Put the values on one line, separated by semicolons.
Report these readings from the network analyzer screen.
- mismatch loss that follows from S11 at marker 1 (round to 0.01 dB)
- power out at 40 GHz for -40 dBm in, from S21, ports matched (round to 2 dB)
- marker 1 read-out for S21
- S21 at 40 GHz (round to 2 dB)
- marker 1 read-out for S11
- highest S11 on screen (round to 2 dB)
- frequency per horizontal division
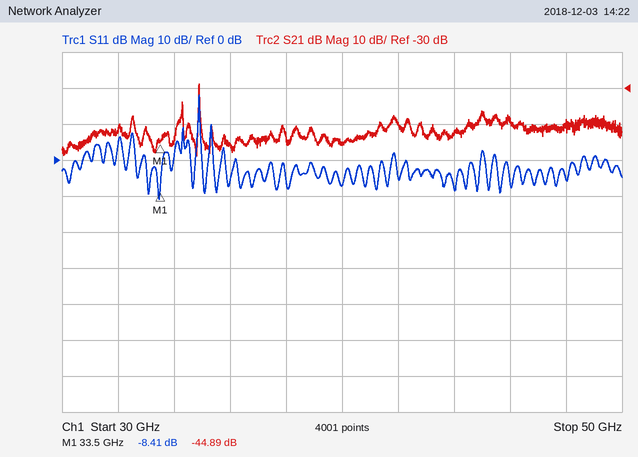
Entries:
0.68 dB; -86 dBm; -44.89 dB; -46 dB; -8.41 dB; 18 dB; 2 GHz
